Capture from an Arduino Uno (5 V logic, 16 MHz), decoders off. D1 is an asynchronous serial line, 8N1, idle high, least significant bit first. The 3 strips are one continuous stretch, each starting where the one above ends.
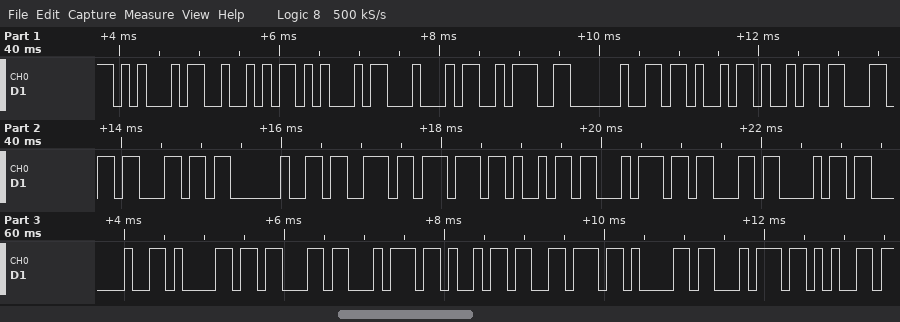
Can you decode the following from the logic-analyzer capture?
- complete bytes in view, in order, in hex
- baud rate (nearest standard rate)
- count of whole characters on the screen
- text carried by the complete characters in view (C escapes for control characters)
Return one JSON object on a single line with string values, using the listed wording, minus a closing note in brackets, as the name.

{"complete bytes in view, in order, in hex": "45 52 45 44 3A 20 4B 69 6C 6C 20 73 77 69 74 63 68 20 61 63 74 69 76 61 74 65", "baud rate": "9600 baud", "count of whole characters on the screen": "26", "text carried by the complete characters in view": "\"ERED: Kill switch activate\""}
